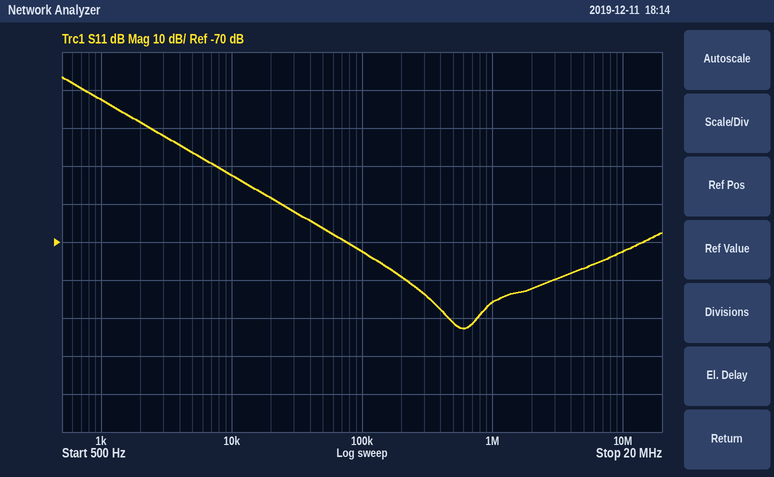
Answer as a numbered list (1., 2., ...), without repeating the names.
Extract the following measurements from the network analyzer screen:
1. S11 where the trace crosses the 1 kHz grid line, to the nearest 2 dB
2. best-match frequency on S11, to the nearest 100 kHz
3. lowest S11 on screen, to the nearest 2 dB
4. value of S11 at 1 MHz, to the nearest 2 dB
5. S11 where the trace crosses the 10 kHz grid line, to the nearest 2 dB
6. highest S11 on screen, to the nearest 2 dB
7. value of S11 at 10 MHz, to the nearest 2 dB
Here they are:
1. -32 dB
2. 600 kHz
3. -92 dB
4. -86 dB
5. -52 dB
6. -26 dB
7. -72 dB
